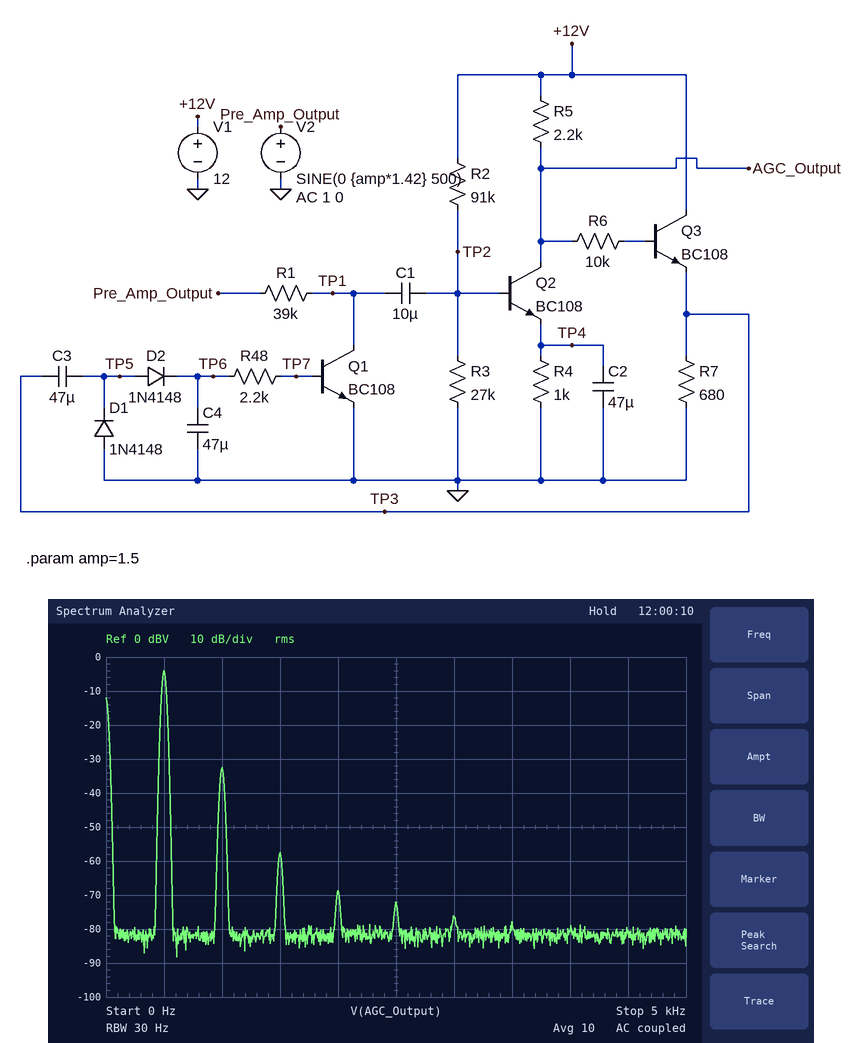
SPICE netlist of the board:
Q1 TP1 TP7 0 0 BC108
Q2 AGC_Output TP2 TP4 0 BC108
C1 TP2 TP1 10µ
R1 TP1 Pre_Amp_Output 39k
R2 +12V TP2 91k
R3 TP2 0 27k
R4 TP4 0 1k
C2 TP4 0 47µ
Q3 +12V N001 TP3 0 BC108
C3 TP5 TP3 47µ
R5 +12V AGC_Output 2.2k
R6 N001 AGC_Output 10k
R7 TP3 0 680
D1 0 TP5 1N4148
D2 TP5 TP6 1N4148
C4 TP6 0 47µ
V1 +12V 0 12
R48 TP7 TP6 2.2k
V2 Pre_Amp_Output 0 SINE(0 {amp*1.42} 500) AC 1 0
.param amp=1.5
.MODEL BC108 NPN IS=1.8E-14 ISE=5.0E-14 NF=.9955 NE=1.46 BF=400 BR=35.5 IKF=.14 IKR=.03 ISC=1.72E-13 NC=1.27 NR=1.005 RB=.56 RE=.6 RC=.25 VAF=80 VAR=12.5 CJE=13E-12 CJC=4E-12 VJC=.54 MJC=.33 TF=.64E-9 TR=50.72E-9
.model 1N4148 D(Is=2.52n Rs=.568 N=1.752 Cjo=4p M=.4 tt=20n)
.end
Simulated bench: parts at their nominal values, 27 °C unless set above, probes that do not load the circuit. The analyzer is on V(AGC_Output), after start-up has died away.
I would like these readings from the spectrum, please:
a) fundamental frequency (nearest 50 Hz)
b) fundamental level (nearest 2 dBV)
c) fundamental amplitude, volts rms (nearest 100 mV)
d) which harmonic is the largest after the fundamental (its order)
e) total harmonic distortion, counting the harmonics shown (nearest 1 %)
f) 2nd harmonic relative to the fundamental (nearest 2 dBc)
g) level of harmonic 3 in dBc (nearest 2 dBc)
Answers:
500 Hz
-4 dBV
600 mV
2
4 %
-28 dBc
-54 dBc
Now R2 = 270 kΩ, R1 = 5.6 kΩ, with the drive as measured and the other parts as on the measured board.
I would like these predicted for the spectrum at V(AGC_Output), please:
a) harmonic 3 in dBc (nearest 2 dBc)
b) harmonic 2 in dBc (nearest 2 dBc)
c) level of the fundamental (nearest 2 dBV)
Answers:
-36 dBc
-14 dBc
-4 dBV
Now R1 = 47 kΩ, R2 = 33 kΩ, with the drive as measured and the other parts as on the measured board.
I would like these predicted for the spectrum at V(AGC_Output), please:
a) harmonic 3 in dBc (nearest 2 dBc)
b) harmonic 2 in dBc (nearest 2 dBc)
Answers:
-18 dBc
-10 dBc
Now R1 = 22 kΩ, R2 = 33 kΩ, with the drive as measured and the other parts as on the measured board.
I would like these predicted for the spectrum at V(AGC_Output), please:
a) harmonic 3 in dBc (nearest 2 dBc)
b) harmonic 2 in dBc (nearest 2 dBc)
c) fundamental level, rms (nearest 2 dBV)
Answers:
-6 dBc
-2 dBc
-8 dBV
